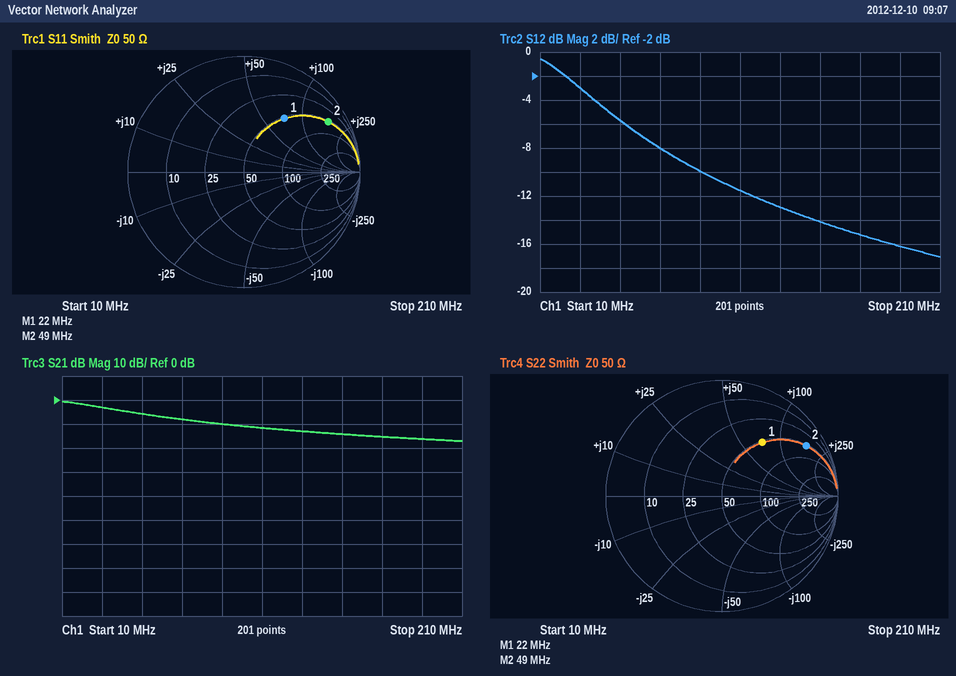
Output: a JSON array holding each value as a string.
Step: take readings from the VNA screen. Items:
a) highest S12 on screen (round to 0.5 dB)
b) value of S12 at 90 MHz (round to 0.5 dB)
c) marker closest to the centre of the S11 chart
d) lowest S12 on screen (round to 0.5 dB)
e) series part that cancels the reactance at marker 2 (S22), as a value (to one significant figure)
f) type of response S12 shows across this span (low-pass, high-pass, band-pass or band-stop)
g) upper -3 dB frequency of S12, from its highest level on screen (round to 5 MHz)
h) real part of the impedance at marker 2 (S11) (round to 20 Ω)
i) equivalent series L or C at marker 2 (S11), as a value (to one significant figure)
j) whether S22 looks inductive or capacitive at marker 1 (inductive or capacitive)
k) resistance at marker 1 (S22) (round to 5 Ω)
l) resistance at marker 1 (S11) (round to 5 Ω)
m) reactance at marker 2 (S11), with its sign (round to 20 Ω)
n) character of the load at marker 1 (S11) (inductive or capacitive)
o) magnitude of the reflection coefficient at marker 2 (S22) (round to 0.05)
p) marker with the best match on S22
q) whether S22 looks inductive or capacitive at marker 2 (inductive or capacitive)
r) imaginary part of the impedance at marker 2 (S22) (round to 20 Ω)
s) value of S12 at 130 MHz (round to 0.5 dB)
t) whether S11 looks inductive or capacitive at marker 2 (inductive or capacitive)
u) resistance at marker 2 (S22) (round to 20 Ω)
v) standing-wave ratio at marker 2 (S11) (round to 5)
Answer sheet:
["-0.5 dB", "-10.0 dB", "marker 1", "-17.0 dB", "20 pF", "low-pass", "35 MHz", "60 Ω", "500 nH", "inductive", "50 Ω", "50 Ω", "+160 Ω", "inductive", "0.85", "marker 1", "inductive", "+160 Ω", "-13.0 dB", "inductive", "60 Ω", "10"]
